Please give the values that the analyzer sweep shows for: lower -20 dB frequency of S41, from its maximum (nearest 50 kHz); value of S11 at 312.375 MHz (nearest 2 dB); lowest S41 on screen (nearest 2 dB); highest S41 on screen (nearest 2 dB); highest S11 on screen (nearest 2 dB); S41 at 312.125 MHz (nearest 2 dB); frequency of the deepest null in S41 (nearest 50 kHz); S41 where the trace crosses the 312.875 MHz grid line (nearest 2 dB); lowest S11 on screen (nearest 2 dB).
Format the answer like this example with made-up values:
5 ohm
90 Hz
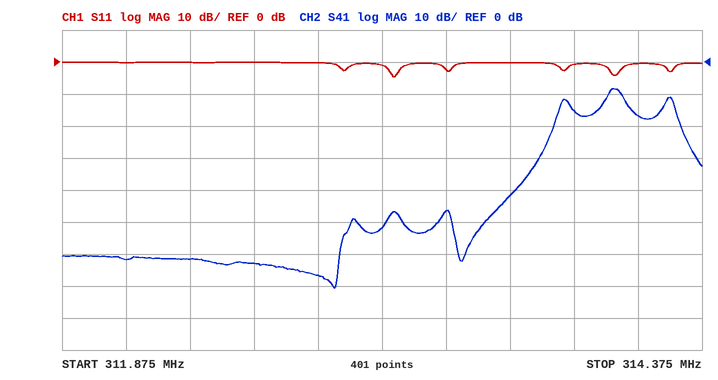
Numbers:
313.75 MHz
0 dB
-70 dB
-8 dB
0 dB
-62 dB
312.95 MHz
-66 dB
-4 dB
